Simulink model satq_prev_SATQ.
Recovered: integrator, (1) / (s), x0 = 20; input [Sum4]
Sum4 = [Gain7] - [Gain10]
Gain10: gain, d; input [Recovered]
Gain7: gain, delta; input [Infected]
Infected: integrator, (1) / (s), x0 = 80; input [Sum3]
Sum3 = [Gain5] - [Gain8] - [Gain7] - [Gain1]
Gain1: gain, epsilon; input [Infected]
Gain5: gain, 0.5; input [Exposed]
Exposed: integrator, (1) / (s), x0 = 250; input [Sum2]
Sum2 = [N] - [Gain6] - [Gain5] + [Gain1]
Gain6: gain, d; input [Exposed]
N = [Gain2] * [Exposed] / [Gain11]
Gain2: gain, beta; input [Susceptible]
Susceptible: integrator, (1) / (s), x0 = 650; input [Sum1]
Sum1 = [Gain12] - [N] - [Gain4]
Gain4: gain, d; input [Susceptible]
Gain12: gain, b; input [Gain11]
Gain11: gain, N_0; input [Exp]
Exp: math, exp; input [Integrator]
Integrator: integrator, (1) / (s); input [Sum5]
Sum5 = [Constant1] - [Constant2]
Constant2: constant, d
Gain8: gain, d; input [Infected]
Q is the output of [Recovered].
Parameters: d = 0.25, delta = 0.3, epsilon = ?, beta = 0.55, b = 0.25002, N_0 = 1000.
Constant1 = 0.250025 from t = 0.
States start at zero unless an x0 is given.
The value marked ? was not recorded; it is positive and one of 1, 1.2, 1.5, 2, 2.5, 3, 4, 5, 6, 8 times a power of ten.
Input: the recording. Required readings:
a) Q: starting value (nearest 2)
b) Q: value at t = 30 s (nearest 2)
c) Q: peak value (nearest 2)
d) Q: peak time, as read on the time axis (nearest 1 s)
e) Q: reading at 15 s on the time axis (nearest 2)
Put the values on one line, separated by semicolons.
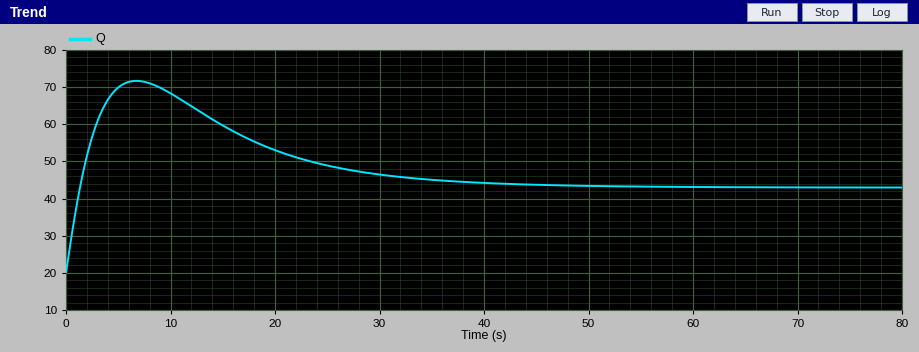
20; 46; 72; 7 s; 60
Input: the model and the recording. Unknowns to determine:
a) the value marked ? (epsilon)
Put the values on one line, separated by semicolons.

0.8
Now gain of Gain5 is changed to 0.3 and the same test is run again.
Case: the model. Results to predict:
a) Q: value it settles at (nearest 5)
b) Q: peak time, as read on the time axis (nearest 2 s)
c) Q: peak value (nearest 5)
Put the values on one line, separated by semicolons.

60; 12 s; 60
